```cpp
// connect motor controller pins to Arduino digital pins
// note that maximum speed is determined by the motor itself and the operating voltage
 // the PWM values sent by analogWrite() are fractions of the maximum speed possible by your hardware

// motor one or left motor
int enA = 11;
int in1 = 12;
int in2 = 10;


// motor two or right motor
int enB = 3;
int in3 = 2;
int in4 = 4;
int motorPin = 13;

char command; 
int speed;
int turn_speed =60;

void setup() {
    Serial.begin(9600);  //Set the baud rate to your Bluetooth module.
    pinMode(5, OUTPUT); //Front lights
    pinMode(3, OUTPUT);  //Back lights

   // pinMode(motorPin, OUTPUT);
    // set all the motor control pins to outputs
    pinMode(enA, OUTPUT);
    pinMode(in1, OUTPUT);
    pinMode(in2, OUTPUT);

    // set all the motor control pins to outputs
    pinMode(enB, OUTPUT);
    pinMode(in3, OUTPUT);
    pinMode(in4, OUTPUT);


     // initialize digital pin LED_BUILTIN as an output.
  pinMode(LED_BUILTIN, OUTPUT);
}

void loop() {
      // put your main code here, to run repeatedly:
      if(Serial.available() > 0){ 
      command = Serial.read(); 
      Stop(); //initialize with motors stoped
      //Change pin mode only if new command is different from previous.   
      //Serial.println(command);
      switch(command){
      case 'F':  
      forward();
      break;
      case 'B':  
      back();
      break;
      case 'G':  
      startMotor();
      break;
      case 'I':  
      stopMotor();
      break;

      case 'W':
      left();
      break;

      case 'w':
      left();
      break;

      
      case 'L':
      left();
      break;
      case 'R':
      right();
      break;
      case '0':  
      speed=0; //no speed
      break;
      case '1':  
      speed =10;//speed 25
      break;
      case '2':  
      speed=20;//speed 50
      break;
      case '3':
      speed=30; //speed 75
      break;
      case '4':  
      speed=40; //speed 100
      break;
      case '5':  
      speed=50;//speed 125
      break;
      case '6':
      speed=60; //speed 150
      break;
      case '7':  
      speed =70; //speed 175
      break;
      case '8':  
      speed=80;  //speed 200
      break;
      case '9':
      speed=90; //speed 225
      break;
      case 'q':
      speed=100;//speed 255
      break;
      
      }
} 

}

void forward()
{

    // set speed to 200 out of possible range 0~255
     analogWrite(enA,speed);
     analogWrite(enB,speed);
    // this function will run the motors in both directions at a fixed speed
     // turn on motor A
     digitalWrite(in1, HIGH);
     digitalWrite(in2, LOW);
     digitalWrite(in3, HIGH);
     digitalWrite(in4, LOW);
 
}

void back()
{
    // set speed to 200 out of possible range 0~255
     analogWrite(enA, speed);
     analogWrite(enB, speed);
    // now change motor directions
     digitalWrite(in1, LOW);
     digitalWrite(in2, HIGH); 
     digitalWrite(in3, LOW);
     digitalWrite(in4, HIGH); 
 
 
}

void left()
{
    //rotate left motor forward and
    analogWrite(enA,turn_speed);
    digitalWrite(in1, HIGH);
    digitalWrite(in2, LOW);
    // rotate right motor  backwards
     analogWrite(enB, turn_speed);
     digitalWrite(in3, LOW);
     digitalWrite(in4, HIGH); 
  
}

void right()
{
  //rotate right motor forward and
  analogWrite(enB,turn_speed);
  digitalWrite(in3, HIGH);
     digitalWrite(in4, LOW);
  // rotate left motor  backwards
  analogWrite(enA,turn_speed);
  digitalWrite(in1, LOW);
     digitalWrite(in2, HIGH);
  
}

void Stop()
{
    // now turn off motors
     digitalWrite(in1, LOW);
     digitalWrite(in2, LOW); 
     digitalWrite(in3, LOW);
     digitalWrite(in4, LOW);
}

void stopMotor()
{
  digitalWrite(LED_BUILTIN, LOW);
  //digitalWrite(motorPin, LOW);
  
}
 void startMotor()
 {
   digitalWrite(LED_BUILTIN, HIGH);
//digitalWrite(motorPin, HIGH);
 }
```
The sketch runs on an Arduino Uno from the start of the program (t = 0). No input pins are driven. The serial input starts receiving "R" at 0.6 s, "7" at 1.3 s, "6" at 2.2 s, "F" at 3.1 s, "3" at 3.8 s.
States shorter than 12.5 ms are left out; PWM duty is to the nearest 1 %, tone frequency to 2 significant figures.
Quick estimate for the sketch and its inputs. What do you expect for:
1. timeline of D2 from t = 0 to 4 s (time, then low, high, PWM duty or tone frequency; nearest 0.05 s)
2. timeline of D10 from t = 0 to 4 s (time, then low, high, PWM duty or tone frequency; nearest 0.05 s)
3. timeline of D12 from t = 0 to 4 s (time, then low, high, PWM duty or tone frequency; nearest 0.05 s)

0 s low; 0.6 s high; 1.3 s low; 3.1 s high; 3.8 s low
0 s low; 0.6 s high; 1.3 s low
0 s low; 3.1 s high; 3.8 s low
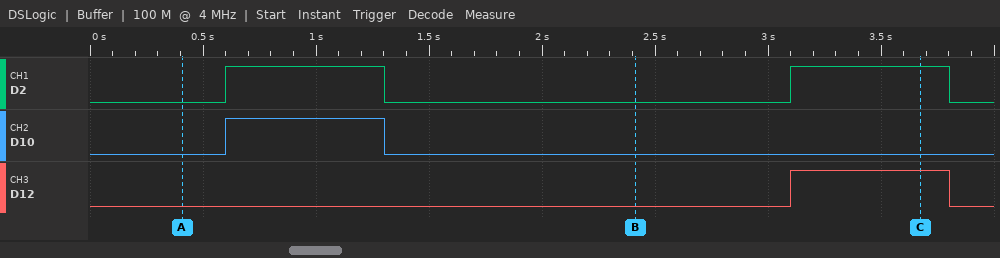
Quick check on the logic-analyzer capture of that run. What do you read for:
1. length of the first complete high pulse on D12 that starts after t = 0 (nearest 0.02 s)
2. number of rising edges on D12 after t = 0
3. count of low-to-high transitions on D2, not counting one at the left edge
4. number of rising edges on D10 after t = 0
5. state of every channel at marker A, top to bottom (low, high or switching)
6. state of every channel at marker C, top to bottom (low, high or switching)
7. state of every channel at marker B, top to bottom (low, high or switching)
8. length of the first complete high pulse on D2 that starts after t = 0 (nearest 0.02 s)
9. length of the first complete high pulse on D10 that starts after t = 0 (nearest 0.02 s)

0.70 s
1
2
1
D2 low, D10 low, D12 low
D2 high, D10 low, D12 high
D2 low, D10 low, D12 low
0.70 s
0.70 s
